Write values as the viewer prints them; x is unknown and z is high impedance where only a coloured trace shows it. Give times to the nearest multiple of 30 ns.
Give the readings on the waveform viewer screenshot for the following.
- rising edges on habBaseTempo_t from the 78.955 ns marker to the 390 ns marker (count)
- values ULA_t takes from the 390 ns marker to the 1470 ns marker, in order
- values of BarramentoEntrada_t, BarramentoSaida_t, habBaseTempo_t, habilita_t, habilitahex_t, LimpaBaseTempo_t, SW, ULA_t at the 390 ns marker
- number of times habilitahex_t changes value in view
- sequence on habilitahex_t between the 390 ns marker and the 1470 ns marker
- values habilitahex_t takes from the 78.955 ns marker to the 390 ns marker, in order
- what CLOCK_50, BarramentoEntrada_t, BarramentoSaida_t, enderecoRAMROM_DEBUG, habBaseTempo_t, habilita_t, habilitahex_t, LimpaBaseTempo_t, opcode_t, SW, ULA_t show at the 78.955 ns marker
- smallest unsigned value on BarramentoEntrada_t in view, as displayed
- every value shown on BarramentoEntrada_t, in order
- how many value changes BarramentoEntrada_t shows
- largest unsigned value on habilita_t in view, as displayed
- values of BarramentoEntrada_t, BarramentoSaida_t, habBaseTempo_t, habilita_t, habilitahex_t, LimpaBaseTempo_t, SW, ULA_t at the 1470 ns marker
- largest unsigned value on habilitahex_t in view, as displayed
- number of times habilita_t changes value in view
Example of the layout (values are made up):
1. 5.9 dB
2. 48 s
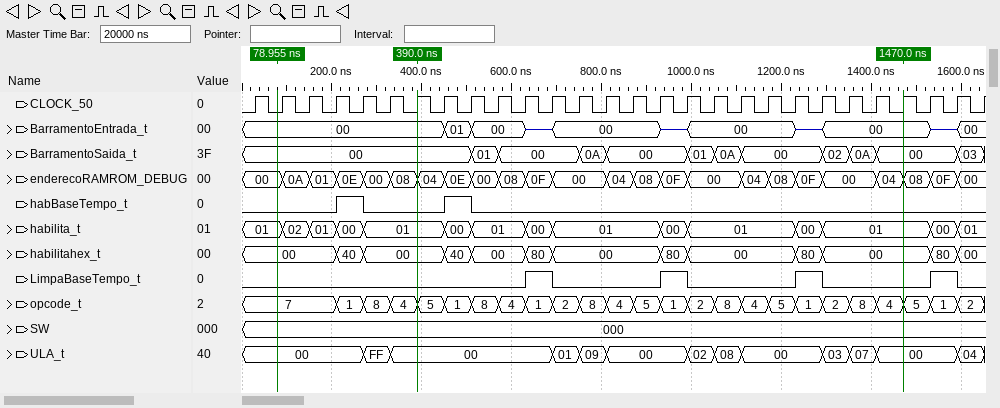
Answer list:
1. 1
2. 00, 01, 09, 00, 02, 08, 00, 03, 07, 00
3. BarramentoEntrada_t=00, BarramentoSaida_t=00, habBaseTempo_t=0, habilita_t=01, habilitahex_t=00, LimpaBaseTempo_t=0, SW=000, ULA_t=00
4. 12
5. 00, 40, 00, 80, 00, 80, 00, 80, 00
6. 00, 40, 00
7. CLOCK_50=0, BarramentoEntrada_t=00, BarramentoSaida_t=00, enderecoRAMROM_DEBUG=00, habBaseTempo_t=0, habilita_t=01, habilitahex_t=00, LimpaBaseTempo_t=0, opcode_t=7, SW=000, ULA_t=00
8. 00
9. 00, 01, 00, z, 00, z, 00, z, 00, z, 00
10. 10
11. 02
12. BarramentoEntrada_t=00, BarramentoSaida_t=00, habBaseTempo_t=0, habilita_t=01, habilitahex_t=00, LimpaBaseTempo_t=0, SW=000, ULA_t=00
13. 80
14. 14
